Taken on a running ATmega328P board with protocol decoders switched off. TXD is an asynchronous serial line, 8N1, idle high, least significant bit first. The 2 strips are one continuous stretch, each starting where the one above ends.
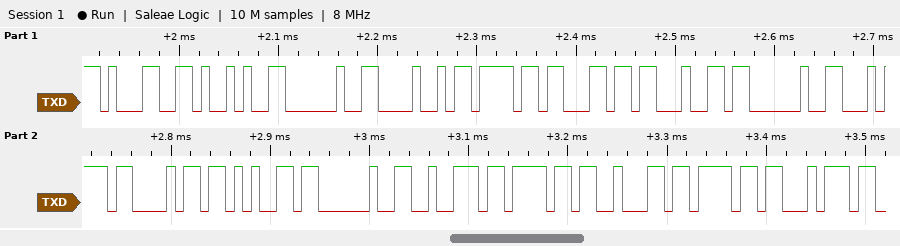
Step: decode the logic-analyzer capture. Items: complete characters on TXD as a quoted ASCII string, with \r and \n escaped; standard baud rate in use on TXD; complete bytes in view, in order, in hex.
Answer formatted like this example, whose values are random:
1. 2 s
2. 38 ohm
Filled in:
1. "1) Hold the robot"
2. 115200 baud
3. 31 29 20 48 6F 6C 64 20 74 68 65 20 72 6F 62 6F 74
